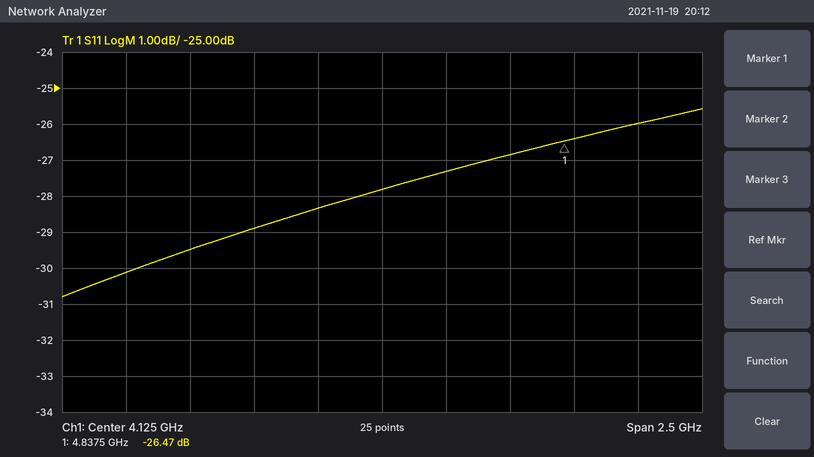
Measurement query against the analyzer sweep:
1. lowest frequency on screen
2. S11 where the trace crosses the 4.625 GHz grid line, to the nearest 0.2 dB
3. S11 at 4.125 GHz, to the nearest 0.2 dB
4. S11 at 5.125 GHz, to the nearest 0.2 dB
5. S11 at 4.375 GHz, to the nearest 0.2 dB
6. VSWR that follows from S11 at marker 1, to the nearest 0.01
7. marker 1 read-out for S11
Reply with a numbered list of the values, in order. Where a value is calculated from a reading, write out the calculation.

1. 2.875 GHz
2. -26.8 dB
3. -27.8 dB
4. -26.0 dB
5. -27.4 dB
6. (1 + 0.0475)/(1 − 0.0475) ≈ 1.10
7. -26.47 dB
